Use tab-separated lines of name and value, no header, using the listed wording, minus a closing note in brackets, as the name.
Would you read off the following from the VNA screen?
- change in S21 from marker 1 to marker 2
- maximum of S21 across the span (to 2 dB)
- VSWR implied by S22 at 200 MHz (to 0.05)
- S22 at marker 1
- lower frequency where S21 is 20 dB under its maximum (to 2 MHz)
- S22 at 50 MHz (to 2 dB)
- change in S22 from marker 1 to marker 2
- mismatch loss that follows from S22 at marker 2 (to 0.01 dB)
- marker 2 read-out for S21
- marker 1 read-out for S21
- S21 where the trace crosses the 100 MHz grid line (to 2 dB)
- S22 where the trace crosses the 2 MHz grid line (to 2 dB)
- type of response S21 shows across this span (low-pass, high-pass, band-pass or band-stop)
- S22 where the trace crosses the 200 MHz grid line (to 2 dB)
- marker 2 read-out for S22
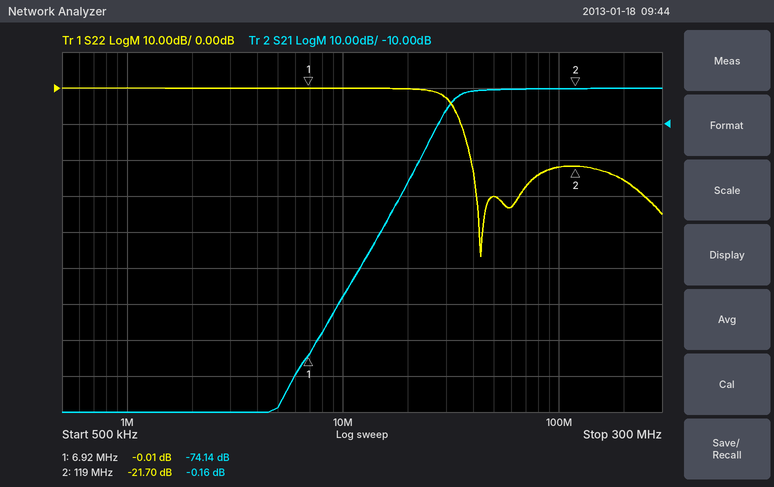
change in S21 from marker 1 to marker 2	73.98 dB
maximum of S21 across the span	0 dB
VSWR implied by S22 at 200 MHz	1.10
S22 at marker 1	-0.01 dB
lower frequency where S21 is 20 dB under its maximum	22 MHz
S22 at 50 MHz	-30 dB
change in S22 from marker 1 to marker 2	-21.69 dB
mismatch loss that follows from S22 at marker 2	0.03 dB
marker 2 read-out for S21	-0.16 dB
marker 1 read-out for S21	-74.14 dB
S21 where the trace crosses the 100 MHz grid line	0 dB
S22 where the trace crosses the 2 MHz grid line	0 dB
type of response S21 shows across this span	high-pass
S22 where the trace crosses the 200 MHz grid line	-26 dB
marker 2 read-out for S22	-21.70 dB
